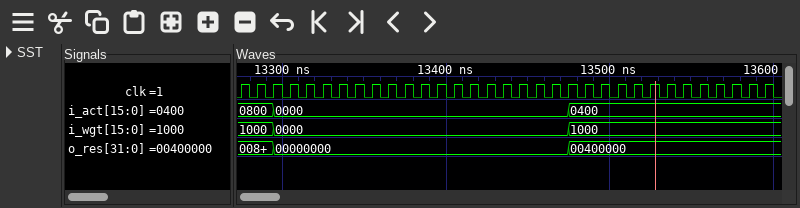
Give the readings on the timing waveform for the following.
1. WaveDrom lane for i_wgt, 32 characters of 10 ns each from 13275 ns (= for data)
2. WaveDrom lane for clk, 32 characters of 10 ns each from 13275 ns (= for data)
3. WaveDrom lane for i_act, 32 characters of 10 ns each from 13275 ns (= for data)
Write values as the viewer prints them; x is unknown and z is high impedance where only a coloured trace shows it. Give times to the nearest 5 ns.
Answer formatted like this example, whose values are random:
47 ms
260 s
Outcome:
{name: 'i_wgt', wave: '=.=.................=...........', data: '1000 0000 1000'}
{name: 'clk', wave: 'p...............................'}
{name: 'i_act', wave: '=.=.................=...........', data: '0800 0000 0400'}
